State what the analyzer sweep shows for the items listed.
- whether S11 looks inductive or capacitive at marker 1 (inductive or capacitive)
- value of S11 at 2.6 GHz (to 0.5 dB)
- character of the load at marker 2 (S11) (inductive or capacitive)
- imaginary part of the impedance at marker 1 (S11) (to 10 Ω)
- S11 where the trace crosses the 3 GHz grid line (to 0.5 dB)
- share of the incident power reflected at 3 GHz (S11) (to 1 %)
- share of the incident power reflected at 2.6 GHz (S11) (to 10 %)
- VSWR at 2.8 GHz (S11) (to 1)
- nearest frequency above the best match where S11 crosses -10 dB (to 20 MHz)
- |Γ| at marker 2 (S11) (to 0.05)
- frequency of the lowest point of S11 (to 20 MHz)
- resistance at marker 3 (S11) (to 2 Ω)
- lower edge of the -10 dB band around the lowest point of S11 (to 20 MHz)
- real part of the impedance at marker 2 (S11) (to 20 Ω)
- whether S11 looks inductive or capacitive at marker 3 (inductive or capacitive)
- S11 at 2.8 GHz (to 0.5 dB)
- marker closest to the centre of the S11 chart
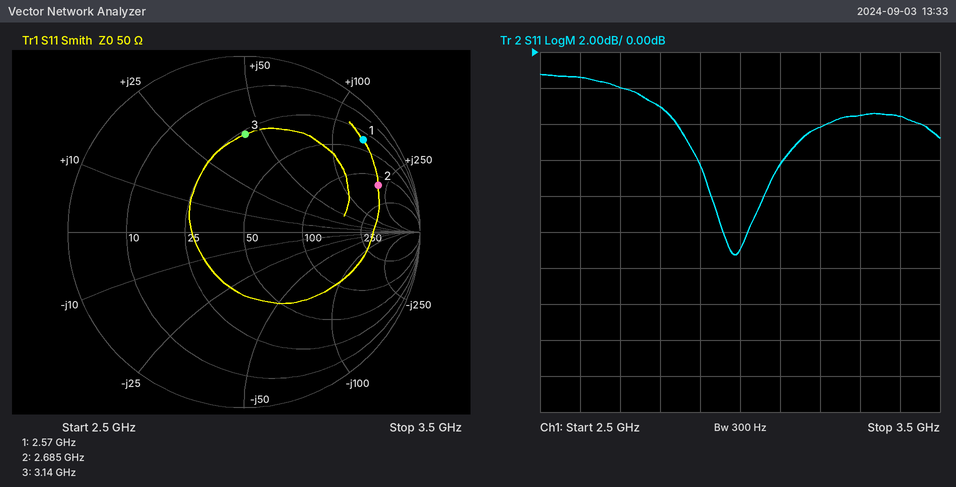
inductive
-1.5 dB
inductive
+140 Ω
-11.0 dB
8 %
70 %
6
3.02 GHz
0.80
2.98 GHz
26 Ω
2.96 GHz
140 Ω
inductive
-3.0 dB
marker 3
